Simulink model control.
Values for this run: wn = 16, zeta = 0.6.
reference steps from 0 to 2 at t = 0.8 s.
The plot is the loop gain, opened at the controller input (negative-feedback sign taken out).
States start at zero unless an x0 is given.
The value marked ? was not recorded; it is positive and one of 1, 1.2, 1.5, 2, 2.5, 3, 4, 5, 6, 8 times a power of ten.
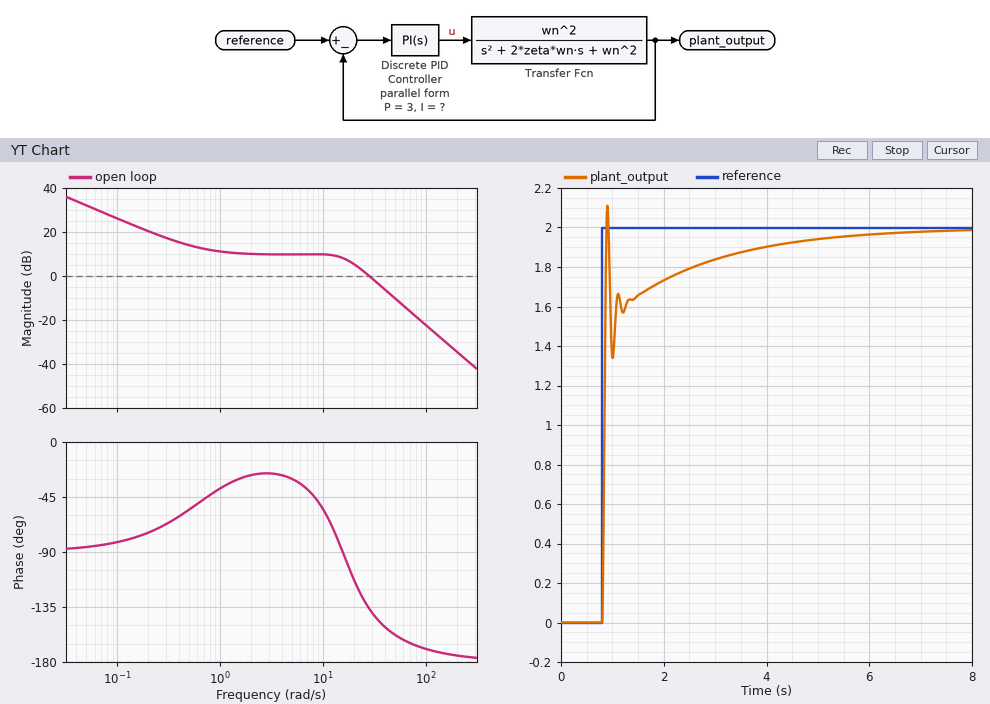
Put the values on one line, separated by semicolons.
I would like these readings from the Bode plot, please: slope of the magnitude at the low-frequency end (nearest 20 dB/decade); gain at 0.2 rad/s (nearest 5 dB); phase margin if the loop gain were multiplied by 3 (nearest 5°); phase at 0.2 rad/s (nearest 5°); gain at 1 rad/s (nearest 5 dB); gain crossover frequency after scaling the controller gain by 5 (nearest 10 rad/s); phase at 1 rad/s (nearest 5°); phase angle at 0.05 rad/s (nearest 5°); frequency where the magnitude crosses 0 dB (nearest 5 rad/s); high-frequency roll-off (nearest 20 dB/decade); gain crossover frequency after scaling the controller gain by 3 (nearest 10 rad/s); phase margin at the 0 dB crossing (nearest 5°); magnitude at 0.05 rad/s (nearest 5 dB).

-20 dB/decade; 20 dB; 25°; -75°; 10 dB; 60 rad/s; -40°; -85°; 30 rad/s; -40 dB/decade; 50 rad/s; 45°; 30 dB
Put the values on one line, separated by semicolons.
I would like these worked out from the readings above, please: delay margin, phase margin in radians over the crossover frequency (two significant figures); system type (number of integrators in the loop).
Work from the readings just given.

0.026 s; 1
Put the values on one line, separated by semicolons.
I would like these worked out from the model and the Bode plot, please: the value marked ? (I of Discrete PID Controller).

2
